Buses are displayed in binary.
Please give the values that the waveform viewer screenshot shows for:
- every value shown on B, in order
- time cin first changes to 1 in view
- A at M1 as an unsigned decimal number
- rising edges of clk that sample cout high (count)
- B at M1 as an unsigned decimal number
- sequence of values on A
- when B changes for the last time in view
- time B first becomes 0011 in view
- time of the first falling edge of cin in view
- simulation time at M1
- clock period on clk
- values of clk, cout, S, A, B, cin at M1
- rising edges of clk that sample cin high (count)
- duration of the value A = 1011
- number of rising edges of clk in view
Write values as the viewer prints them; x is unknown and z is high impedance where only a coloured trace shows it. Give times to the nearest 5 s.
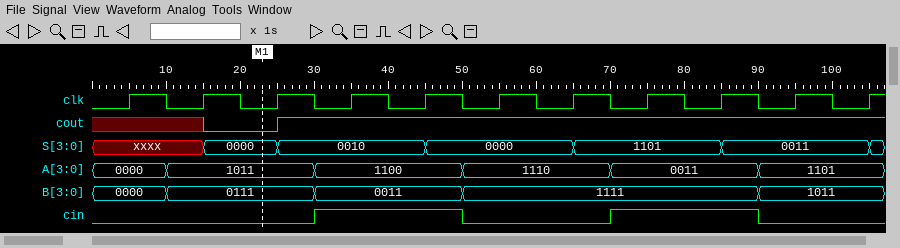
0000, 0111, 0011, 1111, 1011
30 s
11
8
7
0000, 1011, 1100, 1110, 0011, 1101
90 s
30 s
50 s
25 s
10 s
clk=0, cout=0, S=0000, A=1011, B=0111, cin=0
4
20 s
11
